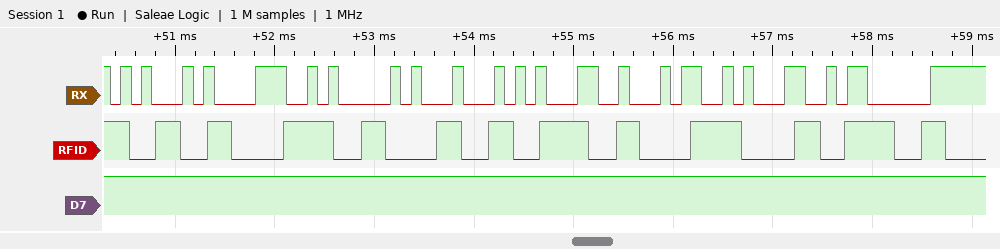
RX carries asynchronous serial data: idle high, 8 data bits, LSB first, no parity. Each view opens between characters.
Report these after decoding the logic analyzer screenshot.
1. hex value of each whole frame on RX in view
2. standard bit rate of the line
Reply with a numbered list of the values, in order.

1. 45, 38, 41, 44, 31, 34, 31, 03
2. 9600 baud
